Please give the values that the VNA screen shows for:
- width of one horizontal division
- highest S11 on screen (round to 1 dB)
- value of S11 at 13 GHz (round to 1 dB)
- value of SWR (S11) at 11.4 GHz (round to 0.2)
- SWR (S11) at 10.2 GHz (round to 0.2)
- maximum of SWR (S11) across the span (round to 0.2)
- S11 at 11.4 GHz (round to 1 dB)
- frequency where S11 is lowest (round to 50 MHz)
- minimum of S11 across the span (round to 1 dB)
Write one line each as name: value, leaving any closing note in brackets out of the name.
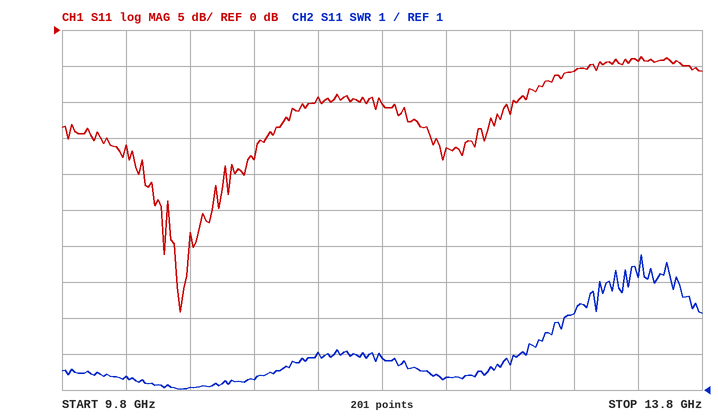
width of one horizontal division: 400 MHz
highest S11 on screen: -4 dB
value of S11 at 13 GHz: -6 dB
value of SWR (S11) at 11.4 GHz: 2.0
SWR (S11) at 10.2 GHz: 1.4
maximum of SWR (S11) across the span: 4.8
S11 at 11.4 GHz: -9 dB
frequency where S11 is lowest: 10.55 GHz
minimum of S11 across the span: -39 dB
